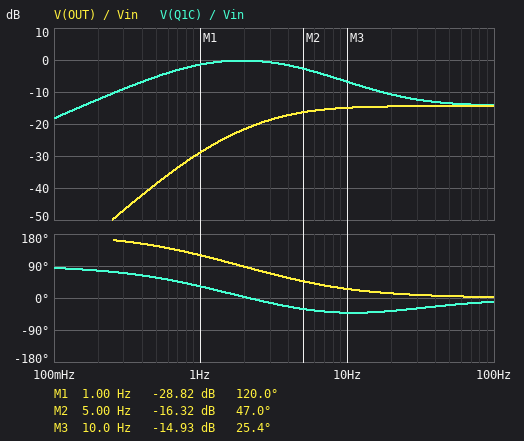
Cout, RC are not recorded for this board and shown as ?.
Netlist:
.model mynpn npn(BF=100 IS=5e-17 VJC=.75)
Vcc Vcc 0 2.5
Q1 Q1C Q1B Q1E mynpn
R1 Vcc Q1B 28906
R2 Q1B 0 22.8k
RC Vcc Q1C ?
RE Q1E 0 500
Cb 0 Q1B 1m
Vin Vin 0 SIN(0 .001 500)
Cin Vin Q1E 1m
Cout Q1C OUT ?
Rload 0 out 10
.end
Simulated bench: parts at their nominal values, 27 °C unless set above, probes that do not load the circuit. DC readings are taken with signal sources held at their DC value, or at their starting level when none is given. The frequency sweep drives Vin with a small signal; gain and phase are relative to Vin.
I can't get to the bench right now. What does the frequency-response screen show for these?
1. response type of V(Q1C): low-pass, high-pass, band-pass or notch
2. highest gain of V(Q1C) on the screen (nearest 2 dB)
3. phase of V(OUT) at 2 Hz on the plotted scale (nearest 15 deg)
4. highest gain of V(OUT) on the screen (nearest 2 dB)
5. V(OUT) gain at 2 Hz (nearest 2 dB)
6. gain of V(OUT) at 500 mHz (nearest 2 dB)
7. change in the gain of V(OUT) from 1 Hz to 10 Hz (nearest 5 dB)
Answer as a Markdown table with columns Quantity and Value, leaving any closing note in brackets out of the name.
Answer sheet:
| Quantity | Value |
|---|---|
| response type of V(Q1C): low-pass, high-pass, band-pass or notch | band-pass |
| highest gain of V(Q1C) on the screen | 0 dB |
| phase of V(OUT) at 2 Hz on the plotted scale | 90 deg |
| highest gain of V(OUT) on the screen | -14 dB |
| V(OUT) gain at 2 Hz | -22 dB |
| gain of V(OUT) at 500 mHz | -38 dB |
| change in the gain of V(OUT) from 1 Hz to 10 Hz | 15 dB |
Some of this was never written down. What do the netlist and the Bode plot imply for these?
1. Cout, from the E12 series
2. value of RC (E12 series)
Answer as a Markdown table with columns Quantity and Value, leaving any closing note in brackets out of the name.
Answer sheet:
| Quantity | Value |
|---|---|
| Cout, from the E12 series | 680 µF |
| value of RC | 220 Ω |
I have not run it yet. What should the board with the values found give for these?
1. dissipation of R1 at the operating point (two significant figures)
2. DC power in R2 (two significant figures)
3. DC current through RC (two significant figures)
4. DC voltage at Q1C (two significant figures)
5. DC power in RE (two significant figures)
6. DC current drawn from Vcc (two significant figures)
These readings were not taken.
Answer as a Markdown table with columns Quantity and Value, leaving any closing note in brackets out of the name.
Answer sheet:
| Quantity | Value |
|---|---|
| dissipation of R1 at the operating point | 74 µW |
| DC power in R2 | 47 µW |
| DC current through RC | 520 µA |
| DC voltage at Q1C | 2.4 V |
| DC power in RE | 140 µW |
| DC current drawn from Vcc | 570 µA |
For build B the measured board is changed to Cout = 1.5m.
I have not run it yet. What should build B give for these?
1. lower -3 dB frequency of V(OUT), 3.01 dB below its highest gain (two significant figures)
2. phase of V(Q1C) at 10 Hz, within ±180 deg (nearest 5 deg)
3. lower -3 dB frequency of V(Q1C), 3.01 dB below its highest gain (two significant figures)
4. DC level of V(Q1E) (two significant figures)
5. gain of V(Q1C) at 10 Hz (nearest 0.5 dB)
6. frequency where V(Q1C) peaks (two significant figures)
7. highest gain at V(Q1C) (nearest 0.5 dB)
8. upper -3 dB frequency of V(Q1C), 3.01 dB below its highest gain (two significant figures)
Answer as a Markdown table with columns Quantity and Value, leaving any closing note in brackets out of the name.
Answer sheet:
| Quantity | Value |
|---|---|
| lower -3 dB frequency of V(OUT), 3.01 dB below its highest gain | 3.6 Hz |
| phase of V(Q1C) at 10 Hz, within ±180 deg | -25 deg |
| lower -3 dB frequency of V(Q1C), 3.01 dB below its highest gain | 380 mHz |
| DC level of V(Q1E) | 260 mV |
| gain of V(Q1C) at 10 Hz | -11.5 dB |
| frequency where V(Q1C) peaks | 1.3 Hz |
| highest gain at V(Q1C) | -6.0 dB |
| upper -3 dB frequency of V(Q1C), 3.01 dB below its highest gain | 5.1 Hz |
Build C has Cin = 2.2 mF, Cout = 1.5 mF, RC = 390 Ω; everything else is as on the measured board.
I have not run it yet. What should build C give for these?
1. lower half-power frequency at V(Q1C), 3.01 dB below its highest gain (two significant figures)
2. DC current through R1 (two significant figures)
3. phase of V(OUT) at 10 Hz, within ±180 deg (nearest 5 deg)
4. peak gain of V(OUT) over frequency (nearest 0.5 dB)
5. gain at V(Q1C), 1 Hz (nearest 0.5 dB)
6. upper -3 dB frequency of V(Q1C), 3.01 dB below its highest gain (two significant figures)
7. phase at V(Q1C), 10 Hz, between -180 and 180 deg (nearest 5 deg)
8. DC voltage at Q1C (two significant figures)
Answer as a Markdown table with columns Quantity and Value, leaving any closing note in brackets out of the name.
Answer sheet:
| Quantity | Value |
|---|---|
| lower half-power frequency at V(Q1C), 3.01 dB below its highest gain | 210 mHz |
| DC current through R1 | 51 µA |
| phase of V(OUT) at 10 Hz, within ±180 deg | 10 deg |
| peak gain of V(OUT) over frequency | -14.0 dB |
| gain at V(Q1C), 1 Hz | 0.5 dB |
| upper -3 dB frequency of V(Q1C), 3.01 dB below its highest gain | 2.2 Hz |
| phase at V(Q1C), 10 Hz, between -180 and 180 deg | -35 deg |
| DC voltage at Q1C | 2.3 V |
